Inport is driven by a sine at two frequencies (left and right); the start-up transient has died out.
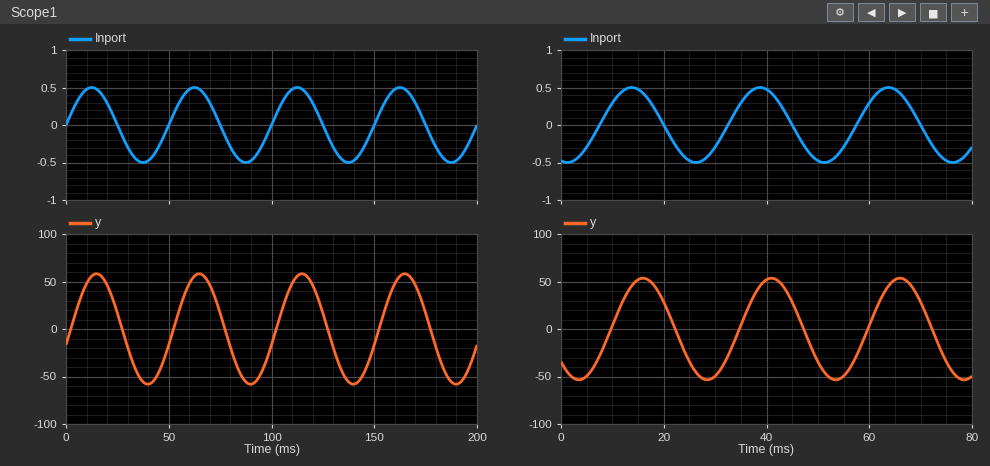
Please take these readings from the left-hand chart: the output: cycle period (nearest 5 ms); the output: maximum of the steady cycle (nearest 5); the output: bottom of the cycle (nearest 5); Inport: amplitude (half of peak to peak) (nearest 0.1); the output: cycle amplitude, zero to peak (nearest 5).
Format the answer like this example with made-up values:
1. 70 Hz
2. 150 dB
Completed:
1. 50 ms
2. 60
3. -60
4. 0.5
5. 60
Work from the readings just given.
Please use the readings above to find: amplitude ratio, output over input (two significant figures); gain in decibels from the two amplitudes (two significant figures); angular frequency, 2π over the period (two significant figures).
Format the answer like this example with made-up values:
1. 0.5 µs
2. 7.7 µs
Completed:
1. 120
2. 42 dB
3. 0.13 rad/ms
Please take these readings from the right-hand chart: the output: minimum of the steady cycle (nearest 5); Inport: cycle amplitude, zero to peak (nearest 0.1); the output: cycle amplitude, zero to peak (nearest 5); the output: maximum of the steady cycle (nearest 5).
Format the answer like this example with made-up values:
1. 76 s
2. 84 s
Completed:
1. -55
2. 0.5
3. 55
4. 55
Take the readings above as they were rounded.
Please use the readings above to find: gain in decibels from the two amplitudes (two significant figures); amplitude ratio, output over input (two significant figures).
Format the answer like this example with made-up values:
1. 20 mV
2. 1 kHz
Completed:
1. 41 dB
2. 110
